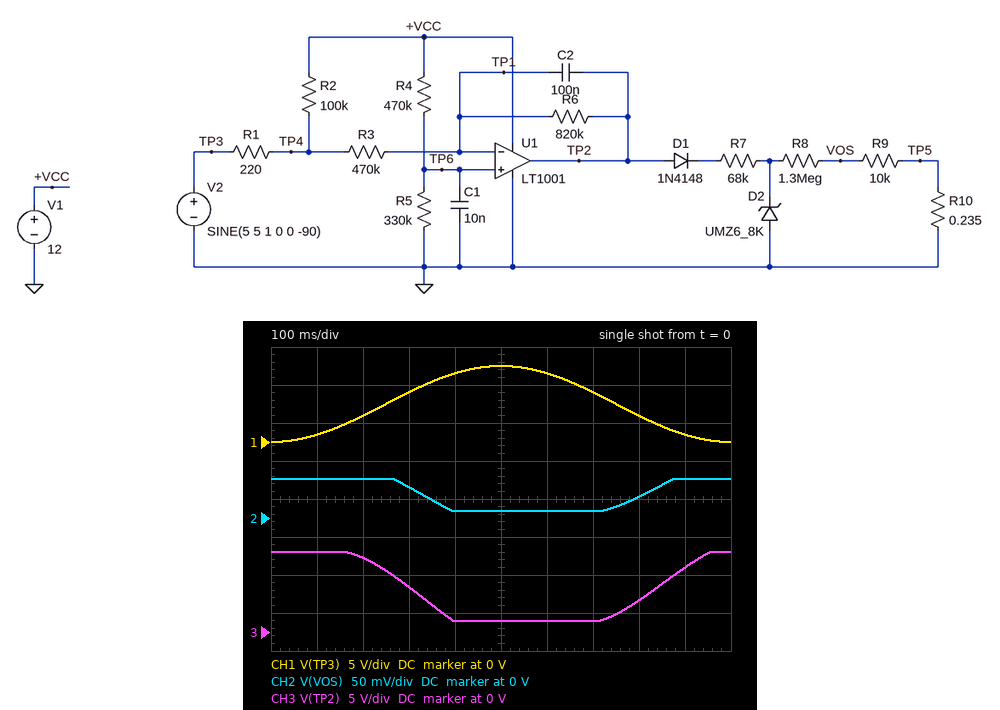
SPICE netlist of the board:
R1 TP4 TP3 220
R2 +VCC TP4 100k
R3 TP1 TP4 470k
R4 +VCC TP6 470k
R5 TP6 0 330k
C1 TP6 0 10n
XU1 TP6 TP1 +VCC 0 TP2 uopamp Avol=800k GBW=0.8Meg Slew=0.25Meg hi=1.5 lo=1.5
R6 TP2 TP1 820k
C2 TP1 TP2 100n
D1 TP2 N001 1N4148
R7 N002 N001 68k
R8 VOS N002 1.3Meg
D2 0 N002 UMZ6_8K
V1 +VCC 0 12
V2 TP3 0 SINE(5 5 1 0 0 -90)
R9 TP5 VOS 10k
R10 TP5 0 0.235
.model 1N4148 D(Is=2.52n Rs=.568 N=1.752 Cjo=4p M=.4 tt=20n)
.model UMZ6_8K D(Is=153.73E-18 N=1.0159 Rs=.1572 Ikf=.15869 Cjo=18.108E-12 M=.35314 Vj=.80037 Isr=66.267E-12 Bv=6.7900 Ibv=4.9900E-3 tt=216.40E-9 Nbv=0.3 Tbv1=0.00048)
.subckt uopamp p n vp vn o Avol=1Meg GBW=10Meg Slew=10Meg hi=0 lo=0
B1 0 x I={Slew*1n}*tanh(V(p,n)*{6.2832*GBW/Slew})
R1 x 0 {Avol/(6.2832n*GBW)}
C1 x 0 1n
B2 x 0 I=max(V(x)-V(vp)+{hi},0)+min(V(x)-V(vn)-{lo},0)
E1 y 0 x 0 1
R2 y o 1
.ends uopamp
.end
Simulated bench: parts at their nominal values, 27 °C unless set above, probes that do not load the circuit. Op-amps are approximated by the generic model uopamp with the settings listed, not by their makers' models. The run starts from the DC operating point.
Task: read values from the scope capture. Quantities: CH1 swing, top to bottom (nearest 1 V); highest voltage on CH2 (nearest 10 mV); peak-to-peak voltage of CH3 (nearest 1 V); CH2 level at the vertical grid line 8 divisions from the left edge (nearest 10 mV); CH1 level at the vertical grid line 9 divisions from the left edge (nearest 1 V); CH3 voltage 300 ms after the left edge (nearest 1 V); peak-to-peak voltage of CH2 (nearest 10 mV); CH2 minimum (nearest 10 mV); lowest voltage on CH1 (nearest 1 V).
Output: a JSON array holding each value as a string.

["10 V", "50 mV", "9 V", "30 mV", "1 V", "6 V", "40 mV", "10 mV", "0 V"]
